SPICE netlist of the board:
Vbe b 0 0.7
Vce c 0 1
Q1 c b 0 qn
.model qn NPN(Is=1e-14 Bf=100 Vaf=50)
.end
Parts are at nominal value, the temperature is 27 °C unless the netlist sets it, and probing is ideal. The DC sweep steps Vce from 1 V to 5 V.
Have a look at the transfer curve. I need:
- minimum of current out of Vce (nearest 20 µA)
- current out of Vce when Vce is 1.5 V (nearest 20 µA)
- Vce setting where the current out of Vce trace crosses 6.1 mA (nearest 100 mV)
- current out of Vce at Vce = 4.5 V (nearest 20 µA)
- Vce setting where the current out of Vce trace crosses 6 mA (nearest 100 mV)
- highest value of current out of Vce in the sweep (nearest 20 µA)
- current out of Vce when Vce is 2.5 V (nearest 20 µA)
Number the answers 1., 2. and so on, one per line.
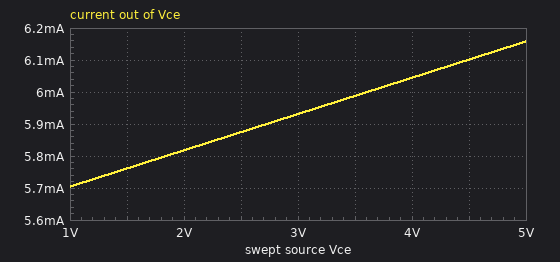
1. 5.70 mA
2. 5.76 mA
3. 4.5 V
4. 6.10 mA
5. 3.6 V
6. 6.16 mA
7. 5.88 mA
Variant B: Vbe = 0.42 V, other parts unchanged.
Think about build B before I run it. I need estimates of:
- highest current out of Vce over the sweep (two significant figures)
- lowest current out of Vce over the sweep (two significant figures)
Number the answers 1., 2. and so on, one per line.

1. 120 nA
2. 110 nA
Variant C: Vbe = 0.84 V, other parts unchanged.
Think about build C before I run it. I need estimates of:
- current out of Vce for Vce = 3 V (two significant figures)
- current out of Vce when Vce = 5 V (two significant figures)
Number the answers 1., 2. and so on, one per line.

1. 1.3 A
2. 1.4 A
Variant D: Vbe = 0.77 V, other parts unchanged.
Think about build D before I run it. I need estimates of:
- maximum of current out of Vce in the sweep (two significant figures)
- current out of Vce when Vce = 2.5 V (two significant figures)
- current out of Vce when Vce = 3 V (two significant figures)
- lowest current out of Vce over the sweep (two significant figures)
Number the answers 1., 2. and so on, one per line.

1. 92 mA
2. 88 mA
3. 89 mA
4. 85 mA
